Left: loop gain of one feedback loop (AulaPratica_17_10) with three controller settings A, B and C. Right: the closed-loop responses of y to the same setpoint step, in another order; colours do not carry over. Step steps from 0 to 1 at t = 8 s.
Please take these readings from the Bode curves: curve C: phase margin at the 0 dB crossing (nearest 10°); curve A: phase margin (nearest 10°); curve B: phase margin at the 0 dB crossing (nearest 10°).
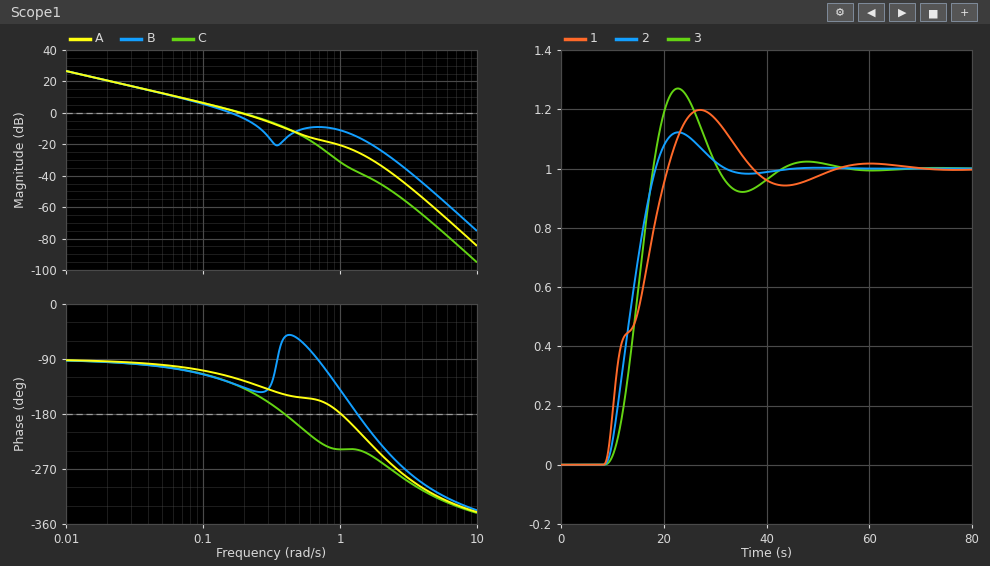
40°
60°
50°
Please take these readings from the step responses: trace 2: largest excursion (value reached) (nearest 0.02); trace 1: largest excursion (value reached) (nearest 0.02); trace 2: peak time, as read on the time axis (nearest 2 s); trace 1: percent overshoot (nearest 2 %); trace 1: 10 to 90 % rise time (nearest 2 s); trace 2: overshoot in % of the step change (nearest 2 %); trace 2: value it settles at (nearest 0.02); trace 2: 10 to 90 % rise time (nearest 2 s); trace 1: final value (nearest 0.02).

1.12
1.20
22 s
20 %
10 s
12 %
1.00
6 s
1.00
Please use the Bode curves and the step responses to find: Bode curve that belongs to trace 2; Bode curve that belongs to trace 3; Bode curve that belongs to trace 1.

A
C
B
